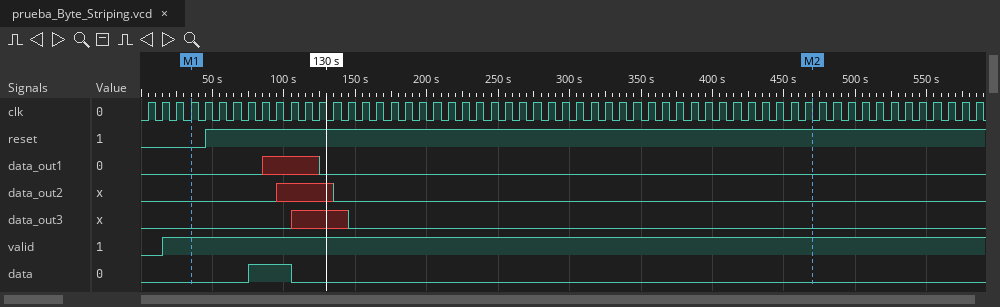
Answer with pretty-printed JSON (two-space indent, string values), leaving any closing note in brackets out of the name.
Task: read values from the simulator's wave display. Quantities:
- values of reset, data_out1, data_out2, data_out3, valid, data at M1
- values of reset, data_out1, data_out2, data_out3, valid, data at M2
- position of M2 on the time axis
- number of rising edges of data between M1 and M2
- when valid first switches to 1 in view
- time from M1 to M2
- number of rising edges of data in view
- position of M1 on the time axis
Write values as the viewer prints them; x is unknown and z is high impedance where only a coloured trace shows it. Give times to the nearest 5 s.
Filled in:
{
  "values of reset, data_out1, data_out2, data_out3, valid, data at M1": "reset=0, data_out1=0, data_out2=0, data_out3=0, valid=1, data=0",
  "values of reset, data_out1, data_out2, data_out3, valid, data at M2": "reset=1, data_out1=0, data_out2=0, data_out3=0, valid=1, data=0",
  "position of M2 on the time axis": "470 s",
  "number of rising edges of data between M1 and M2": "1",
  "when valid first switches to 1 in view": "15 s",
  "time from M1 to M2": "435 s",
  "number of rising edges of data in view": "1",
  "position of M1 on the time axis": "35 s"
}
